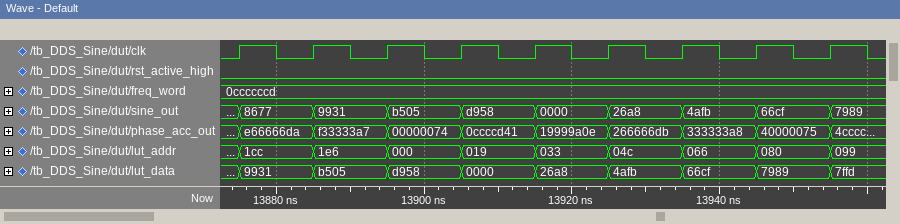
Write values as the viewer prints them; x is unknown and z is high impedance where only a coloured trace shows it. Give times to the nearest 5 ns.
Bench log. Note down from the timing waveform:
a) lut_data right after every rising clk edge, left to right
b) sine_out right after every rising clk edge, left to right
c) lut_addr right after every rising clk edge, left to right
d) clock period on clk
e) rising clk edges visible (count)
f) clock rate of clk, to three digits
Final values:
9931, b505, d958, 0000, 26a8, 4afb, 66cf, 7989, 7ffd
8677, 9931, b505, d958, 0000, 26a8, 4afb, 66cf, 7989
1cc, 1e6, 000, 019, 033, 04c, 066, 080, 099
10 ns
9
100 MHz
